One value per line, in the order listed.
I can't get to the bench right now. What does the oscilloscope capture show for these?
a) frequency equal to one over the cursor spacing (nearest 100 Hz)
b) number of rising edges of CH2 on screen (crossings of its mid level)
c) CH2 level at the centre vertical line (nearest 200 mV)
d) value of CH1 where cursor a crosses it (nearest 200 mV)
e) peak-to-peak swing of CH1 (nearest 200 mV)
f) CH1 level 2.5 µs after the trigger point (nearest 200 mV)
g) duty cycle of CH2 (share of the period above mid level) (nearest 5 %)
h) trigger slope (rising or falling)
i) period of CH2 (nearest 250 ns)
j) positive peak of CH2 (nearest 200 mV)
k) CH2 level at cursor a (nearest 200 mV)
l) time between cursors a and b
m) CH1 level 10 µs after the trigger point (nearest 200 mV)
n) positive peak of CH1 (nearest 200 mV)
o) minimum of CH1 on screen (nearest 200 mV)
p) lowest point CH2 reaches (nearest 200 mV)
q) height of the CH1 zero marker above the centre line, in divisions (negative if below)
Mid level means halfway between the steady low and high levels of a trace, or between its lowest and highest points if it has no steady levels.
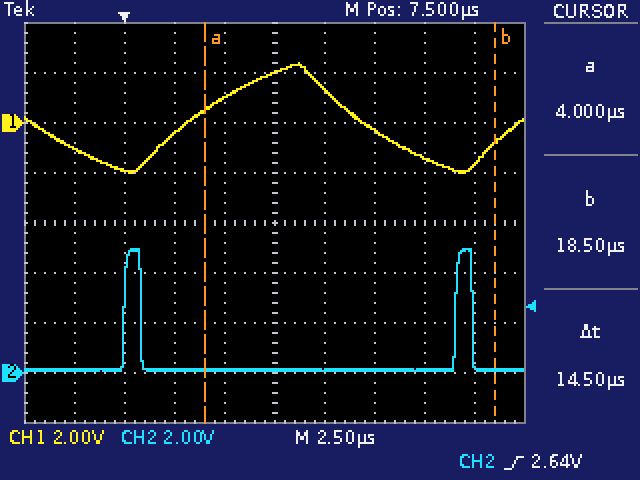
69.0 kHz
2
200 mV
600 mV
4.4 V
-400 mV
5 %
rising
16.50 µs
5.0 V
200 mV
14.5 µs
1.4 V
2.4 V
-2.0 V
0.0 V
+2.0 div
